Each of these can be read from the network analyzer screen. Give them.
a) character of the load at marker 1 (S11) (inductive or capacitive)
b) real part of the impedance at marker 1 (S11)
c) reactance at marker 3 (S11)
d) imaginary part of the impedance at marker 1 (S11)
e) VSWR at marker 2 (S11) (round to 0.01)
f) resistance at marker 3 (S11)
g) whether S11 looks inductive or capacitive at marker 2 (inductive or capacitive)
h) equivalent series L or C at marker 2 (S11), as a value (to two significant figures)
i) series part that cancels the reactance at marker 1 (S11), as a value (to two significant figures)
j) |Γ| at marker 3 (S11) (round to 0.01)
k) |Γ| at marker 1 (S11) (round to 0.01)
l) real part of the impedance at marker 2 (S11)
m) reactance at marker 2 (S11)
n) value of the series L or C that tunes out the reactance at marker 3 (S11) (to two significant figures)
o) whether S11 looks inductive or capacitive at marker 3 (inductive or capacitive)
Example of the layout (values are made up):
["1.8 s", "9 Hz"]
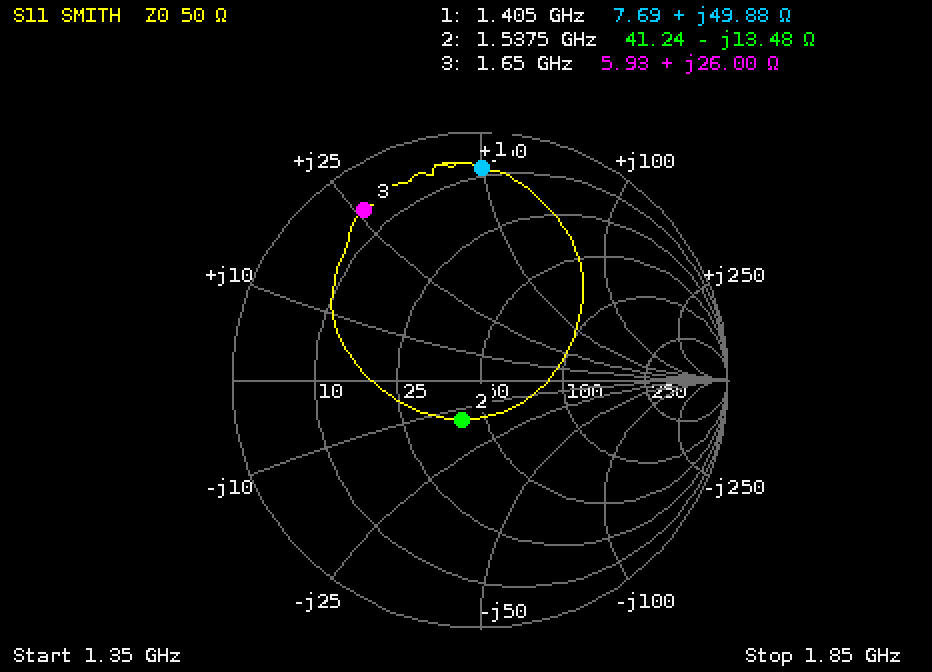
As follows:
["inductive", "7.69 Ω", "+26.00 Ω", "+49.88 Ω", "1.42", "5.93 Ω", "capacitive", "7.7 pF", "2.3 pF", "0.83", "0.86", "41.24 Ω", "-13.48 Ω", "3.7 pF", "inductive"]
